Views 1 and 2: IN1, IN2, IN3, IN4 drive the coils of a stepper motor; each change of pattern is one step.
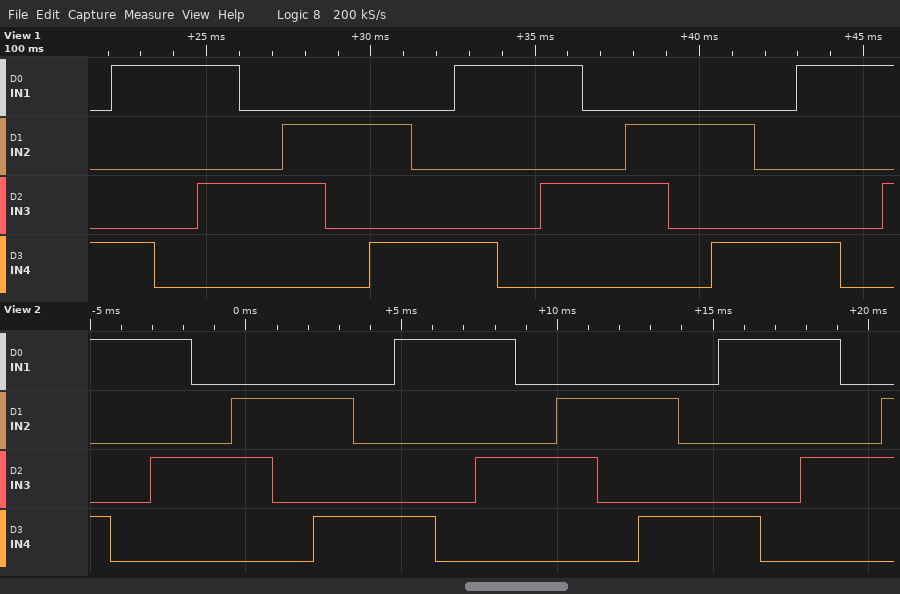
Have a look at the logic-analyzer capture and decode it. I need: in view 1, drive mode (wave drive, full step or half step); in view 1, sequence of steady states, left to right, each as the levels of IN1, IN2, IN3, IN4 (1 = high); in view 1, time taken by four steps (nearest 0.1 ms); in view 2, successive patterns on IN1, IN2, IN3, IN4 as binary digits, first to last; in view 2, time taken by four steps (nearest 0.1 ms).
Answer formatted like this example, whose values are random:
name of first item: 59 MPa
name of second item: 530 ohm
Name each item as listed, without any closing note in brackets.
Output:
in view 1, drive mode: half step
in view 1, sequence of steady states, left to right, each as the levels of IN1, IN2, IN3, IN4: 0001 1001 1000 1010 0010 0110 0100 0101 0001 1001 1000 1010 0010 0110 0100 0101 0001 1001 1000 1010
in view 1, time taken by four steps: 5.2 ms
in view 2, successive patterns on IN1, IN2, IN3, IN4 as binary digits, first to last: 1001 1000 1010 0010 0110 0100 0101 0001 1001 1000 1010 0010 0110 0100 0101 0001 1001 1000 1010 0010 0110
in view 2, time taken by four steps: 5.2 ms
